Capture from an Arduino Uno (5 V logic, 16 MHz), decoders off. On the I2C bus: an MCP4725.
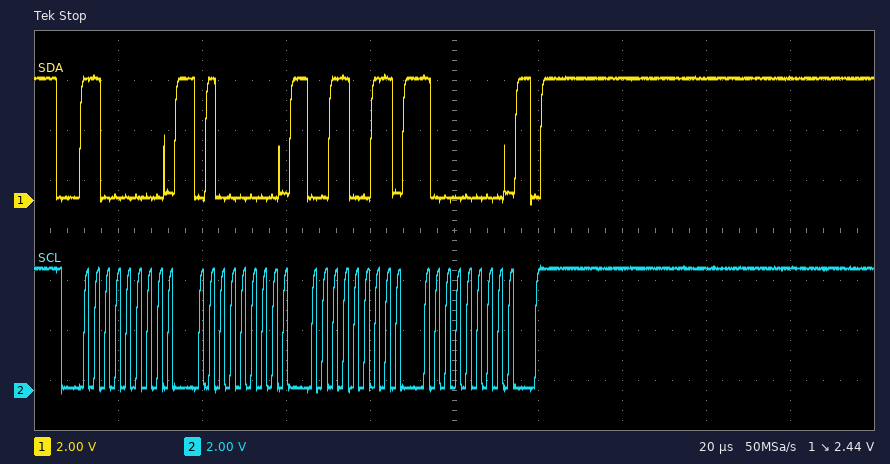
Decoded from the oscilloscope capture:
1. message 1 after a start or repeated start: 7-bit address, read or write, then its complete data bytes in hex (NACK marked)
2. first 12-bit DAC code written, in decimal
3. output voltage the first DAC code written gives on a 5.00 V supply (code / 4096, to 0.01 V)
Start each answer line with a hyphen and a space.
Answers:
- 0x60 write: 40 33 80
- 824
- 1.01 V
